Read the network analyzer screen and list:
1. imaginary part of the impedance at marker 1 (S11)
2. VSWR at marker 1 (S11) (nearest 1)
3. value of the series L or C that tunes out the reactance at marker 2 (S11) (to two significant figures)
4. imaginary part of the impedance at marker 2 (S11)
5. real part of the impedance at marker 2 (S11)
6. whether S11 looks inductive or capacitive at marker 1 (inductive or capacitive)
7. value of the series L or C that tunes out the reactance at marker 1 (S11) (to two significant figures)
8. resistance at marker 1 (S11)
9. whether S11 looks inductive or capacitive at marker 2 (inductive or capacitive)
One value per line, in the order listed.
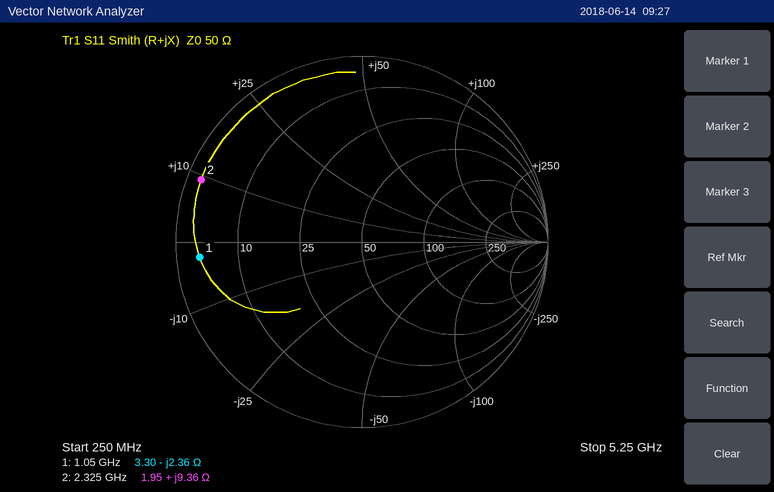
-2.36 Ω
15
7.3 pF
+9.36 Ω
1.95 Ω
capacitive
360 pH
3.30 Ω
inductive
